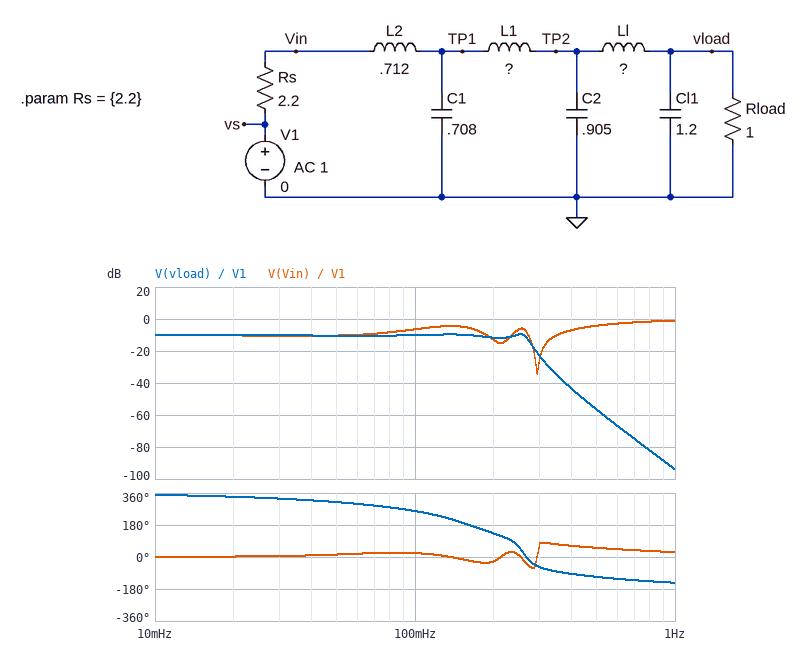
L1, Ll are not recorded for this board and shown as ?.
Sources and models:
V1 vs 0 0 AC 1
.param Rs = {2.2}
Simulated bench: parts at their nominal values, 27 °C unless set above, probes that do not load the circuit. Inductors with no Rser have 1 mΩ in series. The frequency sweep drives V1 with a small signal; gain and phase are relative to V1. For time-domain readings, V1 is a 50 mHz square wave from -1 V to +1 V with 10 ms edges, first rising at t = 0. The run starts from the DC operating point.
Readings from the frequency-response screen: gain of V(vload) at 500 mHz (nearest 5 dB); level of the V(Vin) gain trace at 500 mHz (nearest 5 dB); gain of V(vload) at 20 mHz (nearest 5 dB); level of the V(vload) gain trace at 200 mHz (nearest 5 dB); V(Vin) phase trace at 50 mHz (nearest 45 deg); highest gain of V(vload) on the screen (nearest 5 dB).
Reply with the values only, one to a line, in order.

-55 dB
-5 dB
-10 dB
-10 dB
0 deg
-10 dB
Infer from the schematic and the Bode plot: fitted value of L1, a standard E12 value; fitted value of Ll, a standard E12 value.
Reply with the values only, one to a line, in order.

1.5 H
1 H
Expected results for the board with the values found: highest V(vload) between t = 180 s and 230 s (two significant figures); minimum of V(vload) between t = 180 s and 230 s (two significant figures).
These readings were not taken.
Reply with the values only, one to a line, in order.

420 mV
-420 mV
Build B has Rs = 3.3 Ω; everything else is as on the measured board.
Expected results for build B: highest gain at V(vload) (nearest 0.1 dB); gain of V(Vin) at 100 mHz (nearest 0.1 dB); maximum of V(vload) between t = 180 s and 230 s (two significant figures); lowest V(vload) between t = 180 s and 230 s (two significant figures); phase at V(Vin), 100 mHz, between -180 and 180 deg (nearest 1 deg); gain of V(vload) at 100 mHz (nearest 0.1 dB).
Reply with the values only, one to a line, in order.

-11.2 dB
-8.6 dB
330 mV
-330 mV
26 deg
-12.3 dB
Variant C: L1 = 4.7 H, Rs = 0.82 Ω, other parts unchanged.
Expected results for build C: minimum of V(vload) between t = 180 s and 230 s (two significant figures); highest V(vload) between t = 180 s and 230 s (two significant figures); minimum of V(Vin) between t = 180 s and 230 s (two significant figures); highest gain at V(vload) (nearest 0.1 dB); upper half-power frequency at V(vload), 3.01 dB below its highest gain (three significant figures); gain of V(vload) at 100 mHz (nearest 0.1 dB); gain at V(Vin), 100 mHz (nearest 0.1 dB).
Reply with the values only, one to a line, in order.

-560 mV
560 mV
-1.4 V
-5.2 dB
61.4 mHz
-11.3 dB
-0.6 dB
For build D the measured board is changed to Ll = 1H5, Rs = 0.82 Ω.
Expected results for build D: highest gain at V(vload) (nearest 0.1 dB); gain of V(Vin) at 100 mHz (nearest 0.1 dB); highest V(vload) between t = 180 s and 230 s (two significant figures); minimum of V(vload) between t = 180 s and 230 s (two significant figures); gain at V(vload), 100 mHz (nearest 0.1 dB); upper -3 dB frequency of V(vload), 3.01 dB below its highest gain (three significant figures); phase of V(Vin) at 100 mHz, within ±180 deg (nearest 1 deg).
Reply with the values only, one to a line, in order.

-5.2 dB
-2.5 dB
640 mV
-640 mV
-6.5 dB
218 mHz
5 deg
